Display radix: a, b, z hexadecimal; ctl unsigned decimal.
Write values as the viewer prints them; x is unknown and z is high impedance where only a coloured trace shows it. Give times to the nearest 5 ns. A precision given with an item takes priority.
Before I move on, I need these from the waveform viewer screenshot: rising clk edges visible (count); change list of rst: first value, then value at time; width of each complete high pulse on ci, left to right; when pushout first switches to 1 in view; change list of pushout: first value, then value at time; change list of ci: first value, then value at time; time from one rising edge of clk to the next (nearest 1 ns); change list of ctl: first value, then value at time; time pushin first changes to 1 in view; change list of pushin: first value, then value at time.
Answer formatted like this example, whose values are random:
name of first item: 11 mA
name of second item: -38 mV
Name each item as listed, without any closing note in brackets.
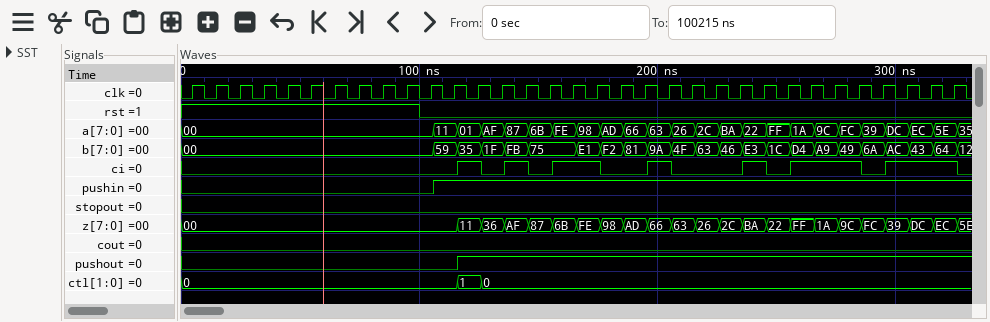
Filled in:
rising clk edges visible: 33
change list of rst: first value, then value at time: 1, 0 at 100 ns
width of each complete high pulse on ci, left to right: 10 ns, 10 ns, 20 ns, 10 ns, 10 ns, 30 ns, 30 ns
when pushout first switches to 1 in view: 115 ns
change list of pushout: first value, then value at time: 0, 1 at 115 ns
change list of ci: first value, then value at time: 0, 1 at 115 ns, 0 at 125 ns, 1 at 135 ns, 0 at 145 ns, 1 at 155 ns, 0 at 175 ns, 1 at 195 ns, 0 at 205 ns, 1 at 235 ns, 0 at 245 ns, 1 at 255 ns, 0 at 285 ns, 1 at 295 ns, 0 at 325 ns
time from one rising edge of clk to the next: 10 ns
change list of ctl: first value, then value at time: 0, 1 at 115 ns, 0 at 125 ns
time pushin first changes to 1 in view: 105 ns
change list of pushin: first value, then value at time: 0, 1 at 105 ns
